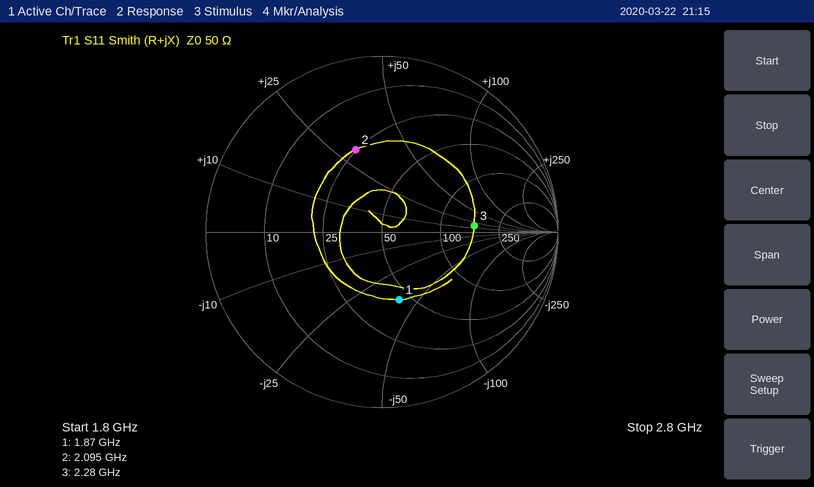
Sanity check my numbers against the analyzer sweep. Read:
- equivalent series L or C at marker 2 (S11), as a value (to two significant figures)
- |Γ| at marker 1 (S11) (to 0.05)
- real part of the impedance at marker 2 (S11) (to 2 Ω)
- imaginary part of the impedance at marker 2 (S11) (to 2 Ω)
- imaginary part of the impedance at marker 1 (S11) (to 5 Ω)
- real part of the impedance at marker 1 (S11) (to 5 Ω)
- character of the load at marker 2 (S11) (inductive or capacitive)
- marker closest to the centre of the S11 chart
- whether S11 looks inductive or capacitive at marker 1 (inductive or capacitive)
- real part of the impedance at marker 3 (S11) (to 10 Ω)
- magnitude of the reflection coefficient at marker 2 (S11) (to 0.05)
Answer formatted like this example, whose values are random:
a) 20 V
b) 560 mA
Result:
a) 2.3 nH
b) 0.40
c) 24 Ω
d) +30 Ω
e) -40 Ω
f) 45 Ω
g) inductive
h) marker 1
i) capacitive
j) 160 Ω
k) 0.50
